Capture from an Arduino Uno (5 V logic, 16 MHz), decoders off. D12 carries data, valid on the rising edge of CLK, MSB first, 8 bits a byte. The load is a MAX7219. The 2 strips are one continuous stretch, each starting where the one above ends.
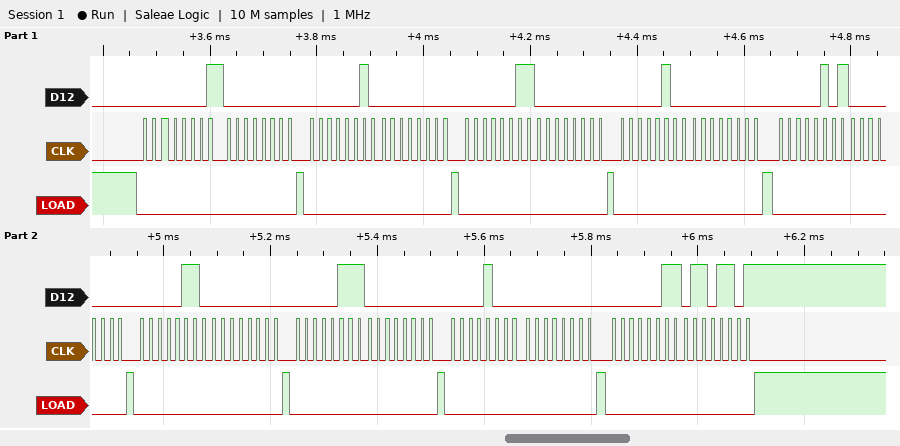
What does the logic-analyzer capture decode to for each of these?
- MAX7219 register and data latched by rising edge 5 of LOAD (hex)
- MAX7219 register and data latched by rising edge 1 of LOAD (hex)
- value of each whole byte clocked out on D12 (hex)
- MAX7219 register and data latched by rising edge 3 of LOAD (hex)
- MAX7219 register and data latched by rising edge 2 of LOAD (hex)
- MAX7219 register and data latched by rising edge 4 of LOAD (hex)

register 0x5, data 0x00
register 0x1, data 0x00
0x01 0x00 0x02 0x00 0x03 0x00 0x04 0x00 0x05 0x00 0x06 0x00 0x07 0x00 0x08 0x00 0x03 0x6D
register 0x3, data 0x00
register 0x2, data 0x00
register 0x4, data 0x00
